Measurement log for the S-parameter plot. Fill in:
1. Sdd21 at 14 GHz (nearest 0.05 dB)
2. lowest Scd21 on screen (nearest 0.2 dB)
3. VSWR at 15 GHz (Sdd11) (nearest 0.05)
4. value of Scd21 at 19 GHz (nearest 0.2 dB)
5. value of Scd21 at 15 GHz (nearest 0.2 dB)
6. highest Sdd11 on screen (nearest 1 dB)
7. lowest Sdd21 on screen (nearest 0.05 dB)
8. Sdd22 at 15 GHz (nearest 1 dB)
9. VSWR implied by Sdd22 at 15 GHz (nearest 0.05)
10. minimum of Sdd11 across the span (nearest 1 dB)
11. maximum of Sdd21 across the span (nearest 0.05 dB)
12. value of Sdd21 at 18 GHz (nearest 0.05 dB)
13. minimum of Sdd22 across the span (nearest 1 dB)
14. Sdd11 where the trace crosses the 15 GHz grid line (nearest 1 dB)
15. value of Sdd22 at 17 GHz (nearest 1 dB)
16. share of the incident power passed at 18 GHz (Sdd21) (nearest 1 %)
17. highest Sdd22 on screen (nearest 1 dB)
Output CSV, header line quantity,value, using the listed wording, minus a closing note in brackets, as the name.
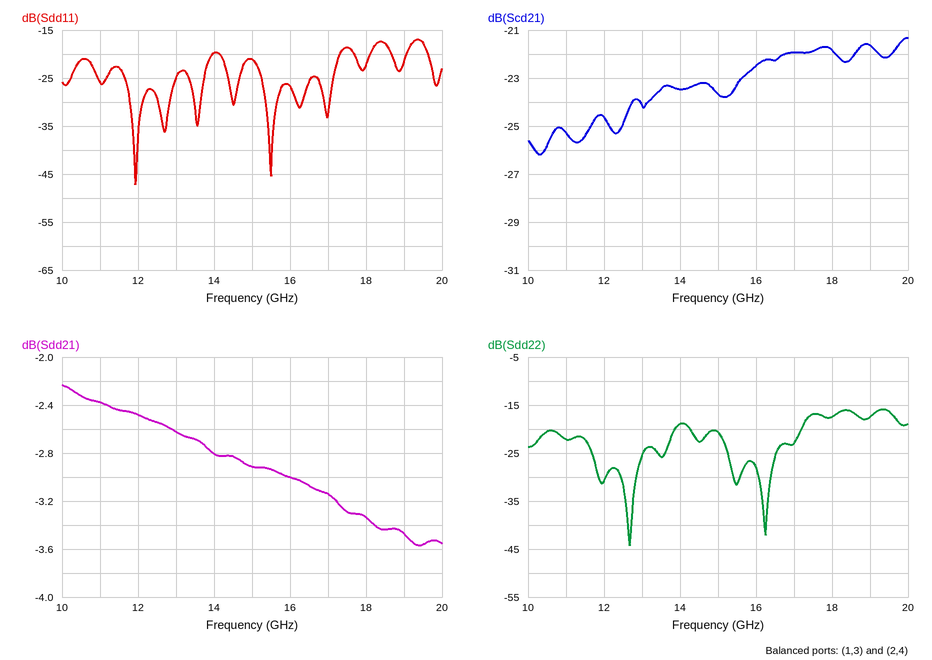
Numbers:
quantity,value
Sdd21 at 14 GHz,-2.80 dB
lowest Scd21 on screen,-26.2 dB
VSWR at 15 GHz (Sdd11),1.20
value of Scd21 at 19 GHz,-21.6 dB
value of Scd21 at 15 GHz,-23.6 dB
highest Sdd11 on screen,-17 dB
lowest Sdd21 on screen,-3.55 dB
Sdd22 at 15 GHz,-21 dB
VSWR implied by Sdd22 at 15 GHz,1.20
minimum of Sdd11 across the span,-47 dB
maximum of Sdd21 across the span,-2.25 dB
value of Sdd21 at 18 GHz,-3.35 dB
minimum of Sdd22 across the span,-44 dB
Sdd11 where the trace crosses the 15 GHz grid line,-21 dB
value of Sdd22 at 17 GHz,-23 dB
share of the incident power passed at 18 GHz (Sdd21),46 %
highest Sdd22 on screen,-16 dB
